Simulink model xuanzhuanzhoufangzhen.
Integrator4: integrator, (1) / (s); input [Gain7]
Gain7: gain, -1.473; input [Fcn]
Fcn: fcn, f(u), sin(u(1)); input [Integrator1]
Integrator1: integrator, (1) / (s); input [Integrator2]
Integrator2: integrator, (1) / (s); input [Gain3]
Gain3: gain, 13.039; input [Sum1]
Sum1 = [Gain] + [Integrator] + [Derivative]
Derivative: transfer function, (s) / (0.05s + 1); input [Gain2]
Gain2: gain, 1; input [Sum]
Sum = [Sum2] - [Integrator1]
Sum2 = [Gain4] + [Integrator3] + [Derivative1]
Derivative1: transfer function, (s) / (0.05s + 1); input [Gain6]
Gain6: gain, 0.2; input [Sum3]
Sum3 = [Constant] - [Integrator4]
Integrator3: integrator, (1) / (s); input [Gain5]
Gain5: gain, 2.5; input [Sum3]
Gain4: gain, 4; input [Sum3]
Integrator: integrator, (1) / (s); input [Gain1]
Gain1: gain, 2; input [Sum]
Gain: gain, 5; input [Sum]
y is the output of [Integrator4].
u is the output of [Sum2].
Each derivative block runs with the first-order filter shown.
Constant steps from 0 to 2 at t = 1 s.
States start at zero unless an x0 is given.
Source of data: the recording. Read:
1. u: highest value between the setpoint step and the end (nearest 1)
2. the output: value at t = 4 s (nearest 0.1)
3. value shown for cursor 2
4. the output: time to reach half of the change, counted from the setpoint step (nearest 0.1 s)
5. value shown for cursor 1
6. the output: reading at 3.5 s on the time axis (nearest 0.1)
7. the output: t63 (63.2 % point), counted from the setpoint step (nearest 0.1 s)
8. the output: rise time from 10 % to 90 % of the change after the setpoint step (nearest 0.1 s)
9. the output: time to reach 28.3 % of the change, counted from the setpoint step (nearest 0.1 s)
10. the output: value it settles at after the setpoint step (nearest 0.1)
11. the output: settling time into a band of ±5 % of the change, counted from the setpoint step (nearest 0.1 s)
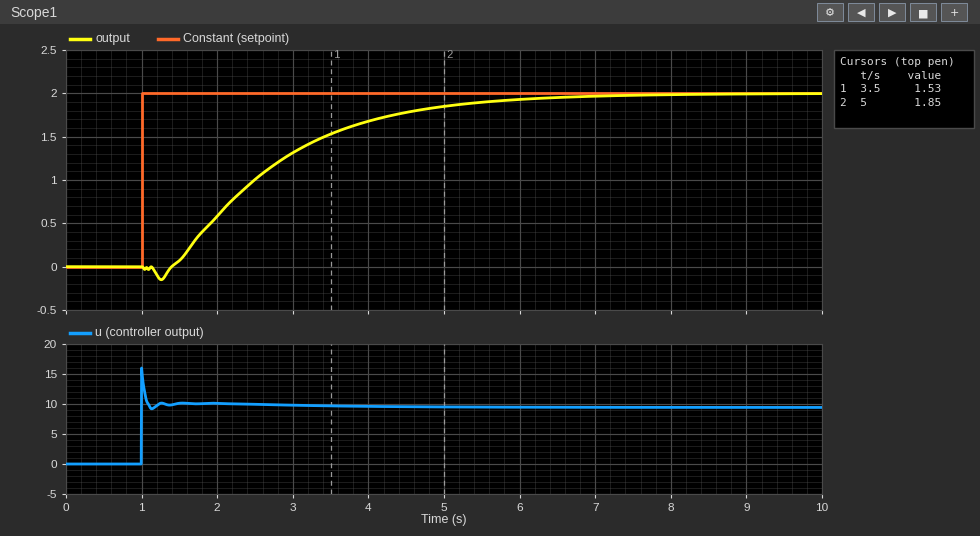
16
1.7
1.85
1.5 s
1.53
1.5
1.9 s
3.0 s
1.0 s
2.0
4.5 s
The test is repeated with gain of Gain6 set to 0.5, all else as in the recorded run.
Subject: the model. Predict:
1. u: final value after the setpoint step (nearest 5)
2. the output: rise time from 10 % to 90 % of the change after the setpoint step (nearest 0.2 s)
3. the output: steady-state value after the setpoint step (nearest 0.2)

10
2.8 s
2.0
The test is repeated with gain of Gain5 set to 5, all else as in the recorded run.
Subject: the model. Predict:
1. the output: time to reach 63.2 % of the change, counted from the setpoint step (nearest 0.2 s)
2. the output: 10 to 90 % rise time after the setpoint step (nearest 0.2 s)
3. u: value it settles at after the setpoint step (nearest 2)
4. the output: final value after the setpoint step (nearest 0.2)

2.4 s
2.0 s
22
2.0
